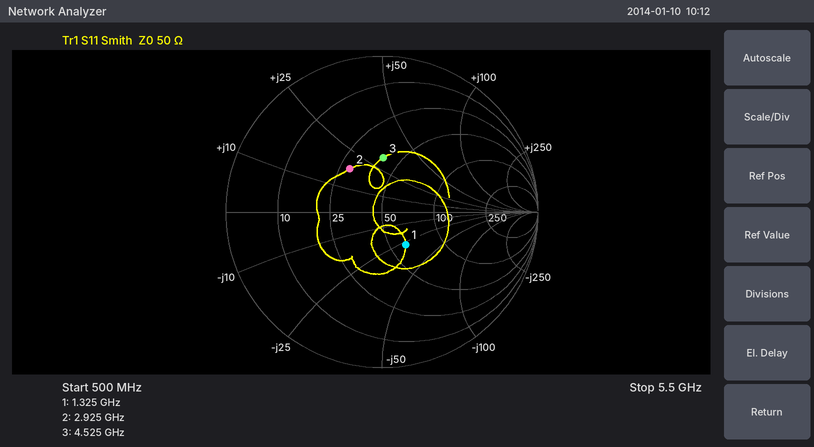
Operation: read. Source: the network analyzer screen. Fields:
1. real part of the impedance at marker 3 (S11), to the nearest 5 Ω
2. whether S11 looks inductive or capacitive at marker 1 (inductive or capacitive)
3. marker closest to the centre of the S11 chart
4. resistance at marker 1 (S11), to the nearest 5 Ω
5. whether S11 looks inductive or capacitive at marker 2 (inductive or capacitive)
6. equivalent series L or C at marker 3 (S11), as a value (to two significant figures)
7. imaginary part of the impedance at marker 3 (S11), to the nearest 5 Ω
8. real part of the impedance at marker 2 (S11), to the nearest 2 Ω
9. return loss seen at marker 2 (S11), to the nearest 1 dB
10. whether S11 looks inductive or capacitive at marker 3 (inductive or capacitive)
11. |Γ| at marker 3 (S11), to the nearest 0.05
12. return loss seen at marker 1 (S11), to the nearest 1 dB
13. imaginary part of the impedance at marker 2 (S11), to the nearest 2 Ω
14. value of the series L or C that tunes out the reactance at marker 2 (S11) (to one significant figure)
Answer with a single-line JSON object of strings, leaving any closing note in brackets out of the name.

{"real part of the impedance at marker 3 (S11), to the nearest 5 Ω": "40 Ω", "whether S11 looks inductive or capacitive at marker 1": "capacitive", "marker closest to the centre of the S11 chart": "marker 1", "resistance at marker 1 (S11), to the nearest 5 Ω": "60 Ω", "whether S11 looks inductive or capacitive at marker 2": "inductive", "equivalent series L or C at marker 3 (S11), as a value": "1.1 nH", "imaginary part of the impedance at marker 3 (S11), to the nearest 5 Ω": "+30 Ω", "real part of the impedance at marker 2 (S11), to the nearest 2 Ω": "28 Ω", "return loss seen at marker 2 (S11), to the nearest 1 dB": "9 dB", "whether S11 looks inductive or capacitive at marker 3": "inductive", "|Γ| at marker 3 (S11), to the nearest 0.05": "0.35", "return loss seen at marker 1 (S11), to the nearest 1 dB": "12 dB", "imaginary part of the impedance at marker 2 (S11), to the nearest 2 Ω": "+18 Ω", "value of the series L or C that tunes out the reactance at marker 2 (S11)": "3 pF"}
